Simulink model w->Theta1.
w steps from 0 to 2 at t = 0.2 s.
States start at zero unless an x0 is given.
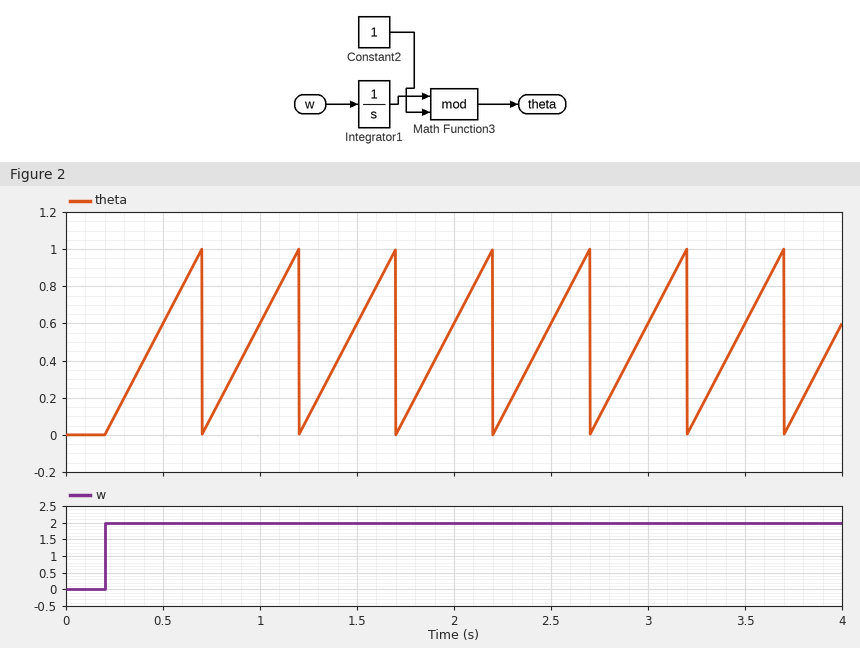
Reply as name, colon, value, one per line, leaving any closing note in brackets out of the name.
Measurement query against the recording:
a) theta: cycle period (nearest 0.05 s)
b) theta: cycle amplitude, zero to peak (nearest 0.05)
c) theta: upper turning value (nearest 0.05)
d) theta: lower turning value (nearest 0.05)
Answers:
theta: cycle period: 0.50 s
theta: cycle amplitude, zero to peak: 0.50
theta: upper turning value: 1.00
theta: lower turning value: 0.00
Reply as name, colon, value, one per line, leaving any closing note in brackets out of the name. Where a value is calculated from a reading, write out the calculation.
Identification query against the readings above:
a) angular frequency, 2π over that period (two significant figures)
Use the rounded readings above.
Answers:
angular frequency, 2π over that period: 2π / 0.5 = 13 rad/s
